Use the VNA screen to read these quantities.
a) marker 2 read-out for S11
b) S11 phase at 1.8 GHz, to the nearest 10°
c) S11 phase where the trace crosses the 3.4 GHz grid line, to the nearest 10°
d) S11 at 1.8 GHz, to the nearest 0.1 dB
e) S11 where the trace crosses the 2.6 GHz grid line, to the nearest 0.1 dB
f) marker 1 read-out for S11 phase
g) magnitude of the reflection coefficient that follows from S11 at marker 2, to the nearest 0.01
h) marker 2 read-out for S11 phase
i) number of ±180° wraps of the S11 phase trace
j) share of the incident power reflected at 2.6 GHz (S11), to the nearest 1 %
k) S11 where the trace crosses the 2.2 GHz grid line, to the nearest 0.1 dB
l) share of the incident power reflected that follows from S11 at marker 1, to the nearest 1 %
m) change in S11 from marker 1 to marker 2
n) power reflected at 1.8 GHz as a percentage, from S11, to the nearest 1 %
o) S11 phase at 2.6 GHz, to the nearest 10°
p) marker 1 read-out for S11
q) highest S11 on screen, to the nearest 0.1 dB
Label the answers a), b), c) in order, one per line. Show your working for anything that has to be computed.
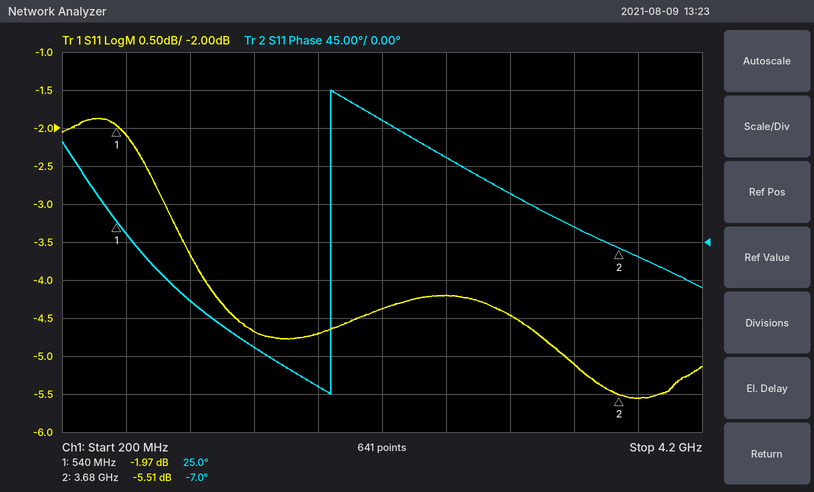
a) -5.51 dB
b) -170°
c) 20°
d) -4.7 dB
e) -4.2 dB
f) 25.0°
g) 10^(-5.51/20) ≈ 0.53
h) -7.0°
i) 1
j) 10^(-4.2/10) ≈ 38 %
k) -4.4 dB
l) 10^(-1.97/10) ≈ 64 %
m) -5.51 − (-1.97) = -3.54 dB
n) 10^(-4.7/10) ≈ 34 %
o) 100°
p) -1.97 dB
q) -1.9 dB
